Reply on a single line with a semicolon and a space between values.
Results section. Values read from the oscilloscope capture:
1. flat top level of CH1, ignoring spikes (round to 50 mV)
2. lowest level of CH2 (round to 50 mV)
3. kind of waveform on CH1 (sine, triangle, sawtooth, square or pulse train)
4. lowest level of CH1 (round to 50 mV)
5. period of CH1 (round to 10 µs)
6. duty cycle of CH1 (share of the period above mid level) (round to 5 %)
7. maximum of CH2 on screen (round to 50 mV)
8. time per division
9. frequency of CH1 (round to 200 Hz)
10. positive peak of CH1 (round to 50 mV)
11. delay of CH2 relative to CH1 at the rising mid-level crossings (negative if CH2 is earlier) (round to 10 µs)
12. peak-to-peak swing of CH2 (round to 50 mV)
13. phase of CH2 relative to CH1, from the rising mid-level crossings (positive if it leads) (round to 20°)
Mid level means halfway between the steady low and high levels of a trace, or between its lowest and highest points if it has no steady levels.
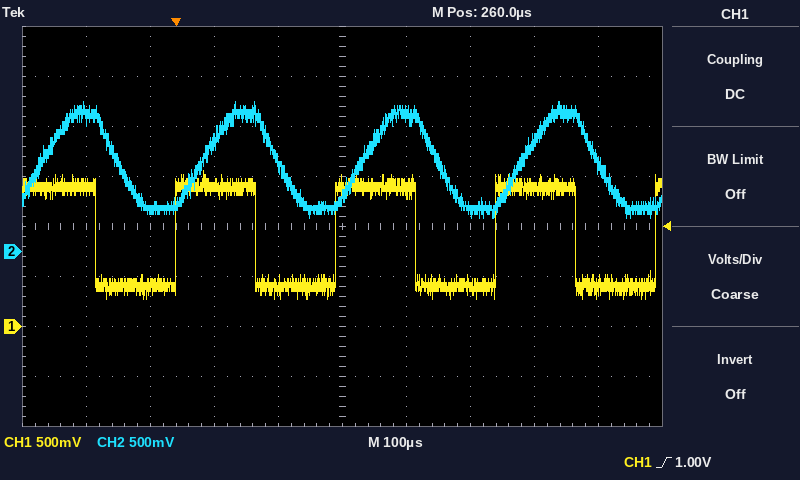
1.40 V; 350 mV; square; 300 mV; 250 µs; 50 %; 1.50 V; 100 µs; 4.0 kHz; 1.55 V; +40 µs; 1.15 V; -60°
